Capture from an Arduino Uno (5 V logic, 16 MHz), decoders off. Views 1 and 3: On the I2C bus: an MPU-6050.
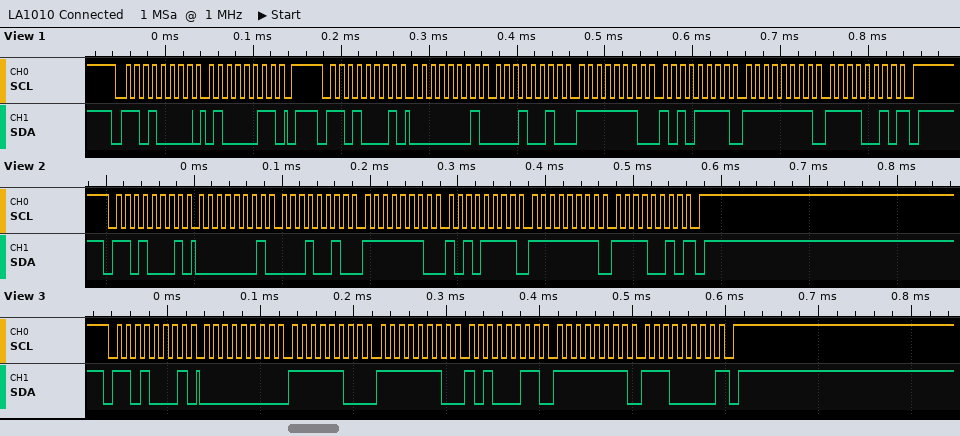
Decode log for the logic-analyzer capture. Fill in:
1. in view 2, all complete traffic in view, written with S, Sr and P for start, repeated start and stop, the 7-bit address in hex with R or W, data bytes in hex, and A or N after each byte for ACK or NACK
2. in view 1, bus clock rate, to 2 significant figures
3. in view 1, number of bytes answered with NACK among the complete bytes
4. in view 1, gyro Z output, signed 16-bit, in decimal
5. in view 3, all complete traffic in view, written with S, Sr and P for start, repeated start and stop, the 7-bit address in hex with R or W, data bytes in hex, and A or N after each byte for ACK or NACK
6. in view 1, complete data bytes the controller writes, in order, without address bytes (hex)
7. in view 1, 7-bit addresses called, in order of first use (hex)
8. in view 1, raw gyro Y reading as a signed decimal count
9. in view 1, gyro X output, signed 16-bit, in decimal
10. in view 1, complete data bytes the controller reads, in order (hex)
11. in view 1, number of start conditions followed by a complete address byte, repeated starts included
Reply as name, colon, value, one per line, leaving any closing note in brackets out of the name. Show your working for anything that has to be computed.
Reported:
in view 2, all complete traffic in view, written with S, Sr and P for start, repeated start and stop, the 7-bit address in hex with R or W, data bytes in hex, and A or N after each byte for ACK or NACK: S 68R A 01 A 12 A FE A AF A FF A F2 N P
in view 1, bus clock rate, to 2 significant figures: 100 kHz
in view 1, number of bytes answered with NACK among the complete bytes: 1
in view 1, gyro Z output, signed 16-bit, in decimal: 0xFFF2 = -14
in view 3, all complete traffic in view, written with S, Sr and P for start, repeated start and stop, the 7-bit address in hex with R or W, data bytes in hex, and A or N after each byte for ACK or NACK: S 68R A 00 A FC A FE A A3 A FF A E0 N P
in view 1, complete data bytes the controller writes, in order, without address bytes: 43
in view 1, 7-bit addresses called, in order of first use: 0x68
in view 1, raw gyro Y reading as a signed decimal count: 0xFEAF = -337
in view 1, gyro X output, signed 16-bit, in decimal: 0x0112 = 274
in view 1, complete data bytes the controller reads, in order: 01 12 FE AF FF F2
in view 1, number of start conditions followed by a complete address byte, repeated starts included: 2
